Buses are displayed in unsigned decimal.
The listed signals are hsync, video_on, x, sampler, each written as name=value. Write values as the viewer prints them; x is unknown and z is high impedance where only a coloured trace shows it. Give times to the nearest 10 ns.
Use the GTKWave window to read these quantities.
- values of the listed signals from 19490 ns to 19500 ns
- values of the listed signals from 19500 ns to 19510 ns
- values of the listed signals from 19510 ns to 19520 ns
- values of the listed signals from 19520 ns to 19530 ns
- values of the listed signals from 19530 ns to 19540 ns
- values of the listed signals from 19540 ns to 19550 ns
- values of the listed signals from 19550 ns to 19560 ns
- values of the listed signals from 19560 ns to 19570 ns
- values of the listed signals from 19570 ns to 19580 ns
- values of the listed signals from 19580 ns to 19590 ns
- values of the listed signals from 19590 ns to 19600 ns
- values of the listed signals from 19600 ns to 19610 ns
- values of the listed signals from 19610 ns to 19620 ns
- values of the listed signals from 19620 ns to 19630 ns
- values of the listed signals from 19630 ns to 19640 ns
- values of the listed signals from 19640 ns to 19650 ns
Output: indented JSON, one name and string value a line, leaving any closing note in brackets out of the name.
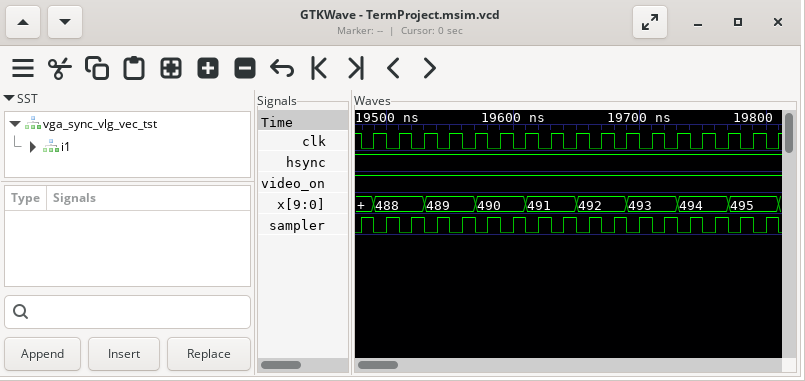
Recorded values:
{
  "values of the listed signals from 19490 ns to 19500 ns": "hsync=1, video_on=1, x=488, sampler=0",
  "values of the listed signals from 19500 ns to 19510 ns": "hsync=1, video_on=1, x=488, sampler=1",
  "values of the listed signals from 19510 ns to 19520 ns": "hsync=1, video_on=1, x=488, sampler=0",
  "values of the listed signals from 19520 ns to 19530 ns": "hsync=1, video_on=1, x=488, sampler=1",
  "values of the listed signals from 19530 ns to 19540 ns": "hsync=1, video_on=1, x=489, sampler=0",
  "values of the listed signals from 19540 ns to 19550 ns": "hsync=1, video_on=1, x=489, sampler=1",
  "values of the listed signals from 19550 ns to 19560 ns": "hsync=1, video_on=1, x=489, sampler=0",
  "values of the listed signals from 19560 ns to 19570 ns": "hsync=1, video_on=1, x=489, sampler=1",
  "values of the listed signals from 19570 ns to 19580 ns": "hsync=1, video_on=1, x=490, sampler=0",
  "values of the listed signals from 19580 ns to 19590 ns": "hsync=1, video_on=1, x=490, sampler=1",
  "values of the listed signals from 19590 ns to 19600 ns": "hsync=1, video_on=1, x=490, sampler=0",
  "values of the listed signals from 19600 ns to 19610 ns": "hsync=1, video_on=1, x=490, sampler=1",
  "values of the listed signals from 19610 ns to 19620 ns": "hsync=1, video_on=1, x=491, sampler=0",
  "values of the listed signals from 19620 ns to 19630 ns": "hsync=1, video_on=1, x=491, sampler=1",
  "values of the listed signals from 19630 ns to 19640 ns": "hsync=1, video_on=1, x=491, sampler=0",
  "values of the listed signals from 19640 ns to 19650 ns": "hsync=1, video_on=1, x=491, sampler=1"
}
